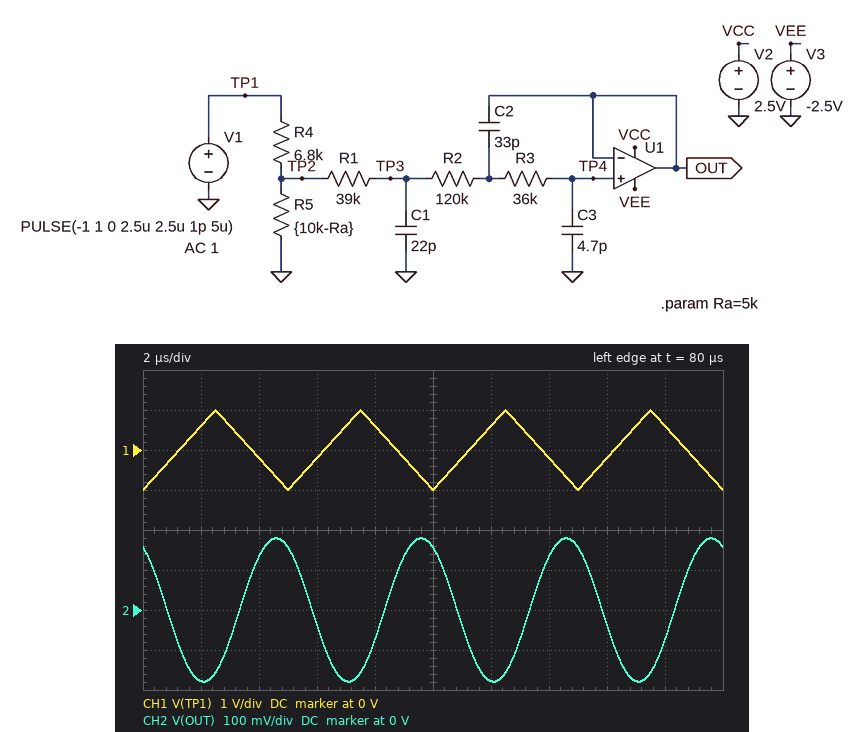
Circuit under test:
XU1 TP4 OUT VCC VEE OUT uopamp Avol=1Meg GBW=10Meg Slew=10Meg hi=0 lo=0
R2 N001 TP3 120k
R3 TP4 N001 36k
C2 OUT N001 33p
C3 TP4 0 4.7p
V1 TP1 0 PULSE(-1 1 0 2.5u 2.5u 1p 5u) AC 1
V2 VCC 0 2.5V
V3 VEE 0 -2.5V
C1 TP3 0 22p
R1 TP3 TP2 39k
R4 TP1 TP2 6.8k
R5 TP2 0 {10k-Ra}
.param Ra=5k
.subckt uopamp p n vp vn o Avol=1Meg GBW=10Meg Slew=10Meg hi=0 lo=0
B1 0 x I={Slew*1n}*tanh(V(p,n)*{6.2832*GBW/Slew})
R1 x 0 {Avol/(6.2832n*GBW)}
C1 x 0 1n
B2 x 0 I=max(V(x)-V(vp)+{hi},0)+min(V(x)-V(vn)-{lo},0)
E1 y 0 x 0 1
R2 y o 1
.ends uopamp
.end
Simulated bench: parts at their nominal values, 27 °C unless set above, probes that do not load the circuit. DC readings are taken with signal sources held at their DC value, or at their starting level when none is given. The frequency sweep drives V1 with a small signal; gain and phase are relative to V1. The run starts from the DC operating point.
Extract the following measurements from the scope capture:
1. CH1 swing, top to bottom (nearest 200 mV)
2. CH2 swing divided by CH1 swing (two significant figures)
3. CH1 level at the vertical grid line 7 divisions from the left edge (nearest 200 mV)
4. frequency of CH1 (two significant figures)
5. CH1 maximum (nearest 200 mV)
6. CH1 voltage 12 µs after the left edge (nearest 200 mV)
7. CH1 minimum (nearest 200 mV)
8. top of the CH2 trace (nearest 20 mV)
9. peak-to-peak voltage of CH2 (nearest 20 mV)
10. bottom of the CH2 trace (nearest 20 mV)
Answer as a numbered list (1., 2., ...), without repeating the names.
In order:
1. 2.0 V
2. 0.18
3. -200 mV
4. 200 kHz
5. 1.0 V
6. 600 mV
7. -1.0 V
8. 180 mV
9. 360 mV
10. -180 mV
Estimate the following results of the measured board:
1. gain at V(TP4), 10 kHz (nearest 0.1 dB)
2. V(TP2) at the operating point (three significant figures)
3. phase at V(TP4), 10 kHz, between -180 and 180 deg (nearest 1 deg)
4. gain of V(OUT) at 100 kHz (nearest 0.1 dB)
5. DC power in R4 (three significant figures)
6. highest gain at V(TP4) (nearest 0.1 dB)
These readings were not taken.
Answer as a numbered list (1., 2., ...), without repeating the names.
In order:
1. -7.5 dB
2. -424 mV
3. -7 deg
4. -7.9 dB
5. 48.8 µW
6. -7.5 dB
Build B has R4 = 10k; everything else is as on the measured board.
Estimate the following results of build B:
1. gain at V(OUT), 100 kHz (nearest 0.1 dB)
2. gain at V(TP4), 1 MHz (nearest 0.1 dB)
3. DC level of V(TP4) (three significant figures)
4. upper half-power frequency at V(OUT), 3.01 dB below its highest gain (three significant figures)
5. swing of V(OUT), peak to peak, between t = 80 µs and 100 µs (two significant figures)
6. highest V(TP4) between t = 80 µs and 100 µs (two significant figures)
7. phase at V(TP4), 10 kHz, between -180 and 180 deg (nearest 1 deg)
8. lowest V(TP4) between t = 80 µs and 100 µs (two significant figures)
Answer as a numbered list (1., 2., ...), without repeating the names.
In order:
1. -10.0 dB
2. -54.2 dB
3. -333 mV
4. 164 kHz
5. 280 mV
6. 140 mV
7. -7 deg
8. -140 mV
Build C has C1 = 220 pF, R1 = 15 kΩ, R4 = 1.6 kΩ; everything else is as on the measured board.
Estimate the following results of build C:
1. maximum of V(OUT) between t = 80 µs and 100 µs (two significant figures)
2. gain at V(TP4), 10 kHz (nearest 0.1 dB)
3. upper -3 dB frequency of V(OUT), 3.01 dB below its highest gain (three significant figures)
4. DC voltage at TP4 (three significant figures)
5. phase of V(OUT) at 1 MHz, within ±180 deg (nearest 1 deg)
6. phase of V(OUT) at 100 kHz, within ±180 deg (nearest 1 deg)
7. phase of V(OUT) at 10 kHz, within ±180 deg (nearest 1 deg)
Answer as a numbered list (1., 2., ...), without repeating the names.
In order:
1. 140 mV
2. -2.6 dB
3. 47.3 kHz
4. -758 mV
5. 97 deg
6. -100 deg
7. -16 deg
